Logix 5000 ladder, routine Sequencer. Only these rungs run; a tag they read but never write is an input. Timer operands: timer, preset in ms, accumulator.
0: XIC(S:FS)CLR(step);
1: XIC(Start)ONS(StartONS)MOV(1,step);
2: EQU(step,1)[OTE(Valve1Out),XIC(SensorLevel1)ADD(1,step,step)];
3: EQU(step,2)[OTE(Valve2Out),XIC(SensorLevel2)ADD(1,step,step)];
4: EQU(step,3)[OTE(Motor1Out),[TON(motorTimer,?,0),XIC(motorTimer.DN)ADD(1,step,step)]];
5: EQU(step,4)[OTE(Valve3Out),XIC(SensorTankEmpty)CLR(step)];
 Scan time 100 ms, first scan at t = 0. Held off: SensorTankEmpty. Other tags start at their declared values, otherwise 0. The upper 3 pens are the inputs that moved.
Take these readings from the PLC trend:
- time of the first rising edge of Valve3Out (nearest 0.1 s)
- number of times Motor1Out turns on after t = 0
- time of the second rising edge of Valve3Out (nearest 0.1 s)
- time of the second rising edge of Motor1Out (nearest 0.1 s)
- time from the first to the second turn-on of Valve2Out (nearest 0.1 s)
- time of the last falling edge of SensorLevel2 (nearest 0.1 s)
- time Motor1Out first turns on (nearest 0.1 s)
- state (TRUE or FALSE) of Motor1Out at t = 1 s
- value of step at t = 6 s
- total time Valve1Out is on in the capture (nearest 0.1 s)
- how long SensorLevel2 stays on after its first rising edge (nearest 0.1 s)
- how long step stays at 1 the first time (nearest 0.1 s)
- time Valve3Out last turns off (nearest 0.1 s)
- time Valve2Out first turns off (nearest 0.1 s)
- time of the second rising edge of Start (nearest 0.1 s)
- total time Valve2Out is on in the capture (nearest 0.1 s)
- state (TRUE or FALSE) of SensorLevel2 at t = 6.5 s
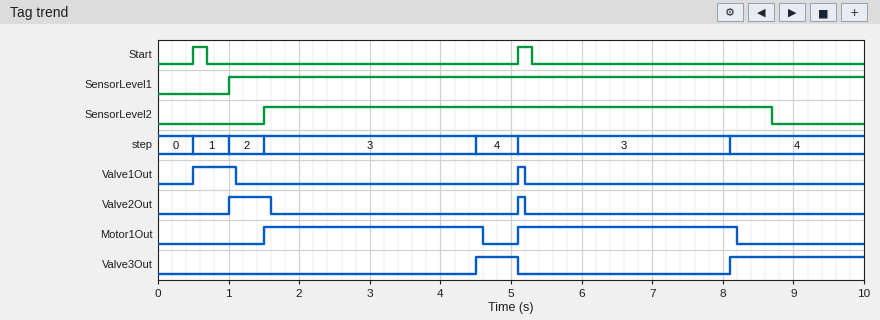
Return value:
4.5 s
2
8.1 s
5.1 s
4.1 s
8.7 s
1.5 s
FALSE
3
0.7 s
7.2 s
0.5 s
5.1 s
1.6 s
5.1 s
0.7 s
TRUE
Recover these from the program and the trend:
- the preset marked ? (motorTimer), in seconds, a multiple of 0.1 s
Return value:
3.0 s
